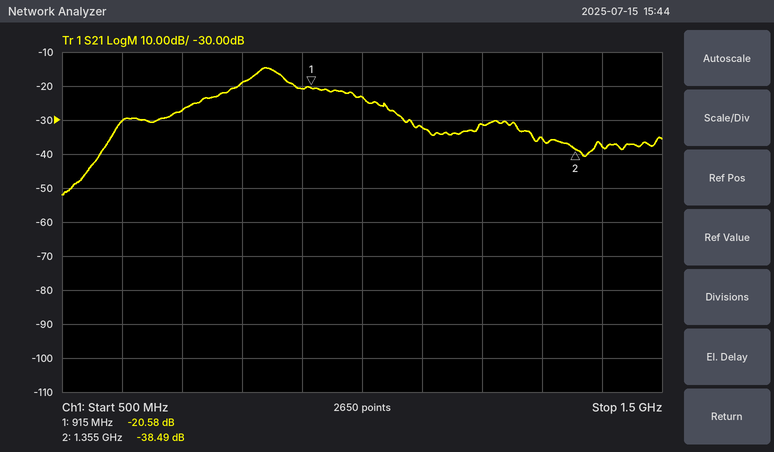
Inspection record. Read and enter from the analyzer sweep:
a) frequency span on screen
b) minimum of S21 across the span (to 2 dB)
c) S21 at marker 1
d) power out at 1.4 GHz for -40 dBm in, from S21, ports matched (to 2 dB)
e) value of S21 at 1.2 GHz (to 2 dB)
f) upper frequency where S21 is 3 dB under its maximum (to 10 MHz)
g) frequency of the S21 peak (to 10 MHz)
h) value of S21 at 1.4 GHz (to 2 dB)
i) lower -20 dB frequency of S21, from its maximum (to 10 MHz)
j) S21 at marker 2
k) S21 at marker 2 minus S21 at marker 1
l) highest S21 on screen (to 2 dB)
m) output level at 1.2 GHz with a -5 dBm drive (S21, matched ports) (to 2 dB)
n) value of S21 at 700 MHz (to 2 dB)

1 GHz
-52 dB
-20.58 dB
-78 dBm
-32 dB
870 MHz
840 MHz
-38 dB
580 MHz
-38.49 dB
-17.91 dB
-14 dB
-36 dBm
-28 dB
